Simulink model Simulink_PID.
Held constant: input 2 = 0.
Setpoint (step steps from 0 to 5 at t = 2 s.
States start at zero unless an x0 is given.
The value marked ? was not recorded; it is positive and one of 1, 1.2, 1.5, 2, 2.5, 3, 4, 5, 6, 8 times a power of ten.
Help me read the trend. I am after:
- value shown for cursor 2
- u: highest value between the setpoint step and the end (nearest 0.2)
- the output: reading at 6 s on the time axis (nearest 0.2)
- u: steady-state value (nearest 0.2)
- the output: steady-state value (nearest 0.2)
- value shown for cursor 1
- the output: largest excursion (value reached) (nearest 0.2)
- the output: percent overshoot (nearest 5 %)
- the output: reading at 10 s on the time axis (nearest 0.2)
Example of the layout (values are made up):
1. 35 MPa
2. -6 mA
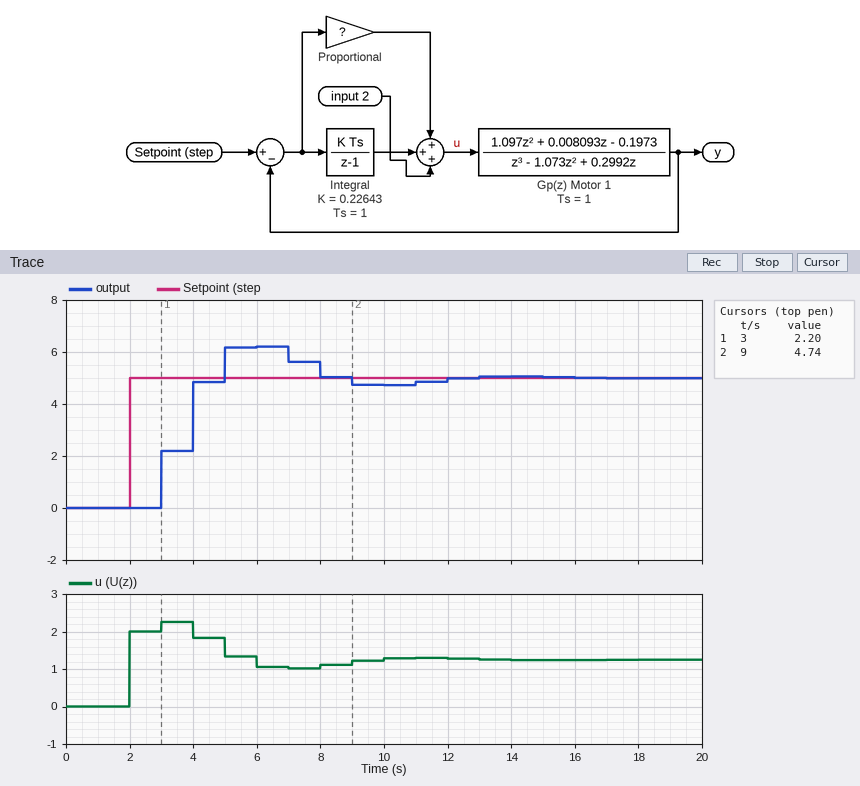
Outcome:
1. 4.74
2. 2.2
3. 6.2
4. 1.2
5. 5.0
6. 2.20
7. 6.2
8. 25 %
9. 4.8
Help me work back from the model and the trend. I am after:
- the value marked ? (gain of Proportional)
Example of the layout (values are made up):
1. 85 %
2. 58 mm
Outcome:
1. 0.4
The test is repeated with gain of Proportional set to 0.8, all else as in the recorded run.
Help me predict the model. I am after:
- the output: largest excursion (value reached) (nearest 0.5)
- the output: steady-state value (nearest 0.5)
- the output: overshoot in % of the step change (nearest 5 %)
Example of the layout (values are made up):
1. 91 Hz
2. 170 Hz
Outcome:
1. 6.5
2. 5.0
3. 30 %
